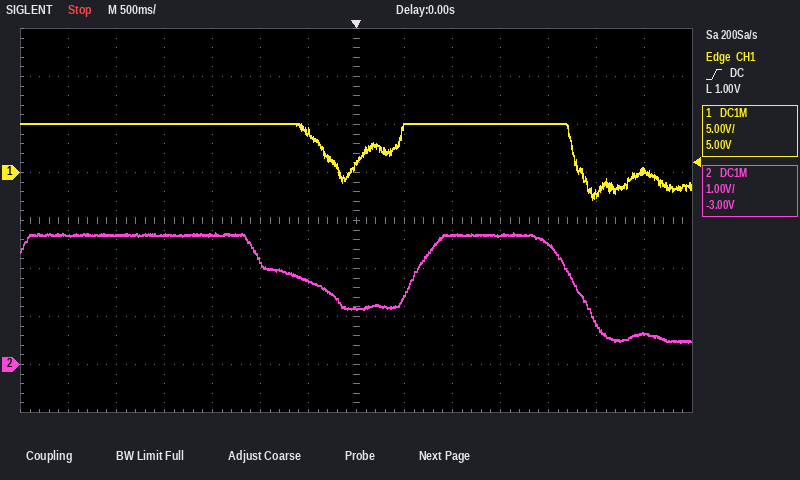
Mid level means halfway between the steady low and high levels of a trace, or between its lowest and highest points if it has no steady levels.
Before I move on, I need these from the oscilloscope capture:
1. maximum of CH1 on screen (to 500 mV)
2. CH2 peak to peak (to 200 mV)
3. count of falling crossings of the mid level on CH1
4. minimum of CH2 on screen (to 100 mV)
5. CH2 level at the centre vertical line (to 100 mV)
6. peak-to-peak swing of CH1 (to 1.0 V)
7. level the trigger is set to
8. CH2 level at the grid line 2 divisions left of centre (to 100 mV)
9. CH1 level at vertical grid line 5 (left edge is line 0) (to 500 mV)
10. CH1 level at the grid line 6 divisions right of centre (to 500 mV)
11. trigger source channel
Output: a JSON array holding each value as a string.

["5.0 V", "2.2 V", "2", "500 mV", "1.2 V", "8.0 V", "1.00 V", "2.1 V", "5.0 V", "0.0 V", "CH1"]
